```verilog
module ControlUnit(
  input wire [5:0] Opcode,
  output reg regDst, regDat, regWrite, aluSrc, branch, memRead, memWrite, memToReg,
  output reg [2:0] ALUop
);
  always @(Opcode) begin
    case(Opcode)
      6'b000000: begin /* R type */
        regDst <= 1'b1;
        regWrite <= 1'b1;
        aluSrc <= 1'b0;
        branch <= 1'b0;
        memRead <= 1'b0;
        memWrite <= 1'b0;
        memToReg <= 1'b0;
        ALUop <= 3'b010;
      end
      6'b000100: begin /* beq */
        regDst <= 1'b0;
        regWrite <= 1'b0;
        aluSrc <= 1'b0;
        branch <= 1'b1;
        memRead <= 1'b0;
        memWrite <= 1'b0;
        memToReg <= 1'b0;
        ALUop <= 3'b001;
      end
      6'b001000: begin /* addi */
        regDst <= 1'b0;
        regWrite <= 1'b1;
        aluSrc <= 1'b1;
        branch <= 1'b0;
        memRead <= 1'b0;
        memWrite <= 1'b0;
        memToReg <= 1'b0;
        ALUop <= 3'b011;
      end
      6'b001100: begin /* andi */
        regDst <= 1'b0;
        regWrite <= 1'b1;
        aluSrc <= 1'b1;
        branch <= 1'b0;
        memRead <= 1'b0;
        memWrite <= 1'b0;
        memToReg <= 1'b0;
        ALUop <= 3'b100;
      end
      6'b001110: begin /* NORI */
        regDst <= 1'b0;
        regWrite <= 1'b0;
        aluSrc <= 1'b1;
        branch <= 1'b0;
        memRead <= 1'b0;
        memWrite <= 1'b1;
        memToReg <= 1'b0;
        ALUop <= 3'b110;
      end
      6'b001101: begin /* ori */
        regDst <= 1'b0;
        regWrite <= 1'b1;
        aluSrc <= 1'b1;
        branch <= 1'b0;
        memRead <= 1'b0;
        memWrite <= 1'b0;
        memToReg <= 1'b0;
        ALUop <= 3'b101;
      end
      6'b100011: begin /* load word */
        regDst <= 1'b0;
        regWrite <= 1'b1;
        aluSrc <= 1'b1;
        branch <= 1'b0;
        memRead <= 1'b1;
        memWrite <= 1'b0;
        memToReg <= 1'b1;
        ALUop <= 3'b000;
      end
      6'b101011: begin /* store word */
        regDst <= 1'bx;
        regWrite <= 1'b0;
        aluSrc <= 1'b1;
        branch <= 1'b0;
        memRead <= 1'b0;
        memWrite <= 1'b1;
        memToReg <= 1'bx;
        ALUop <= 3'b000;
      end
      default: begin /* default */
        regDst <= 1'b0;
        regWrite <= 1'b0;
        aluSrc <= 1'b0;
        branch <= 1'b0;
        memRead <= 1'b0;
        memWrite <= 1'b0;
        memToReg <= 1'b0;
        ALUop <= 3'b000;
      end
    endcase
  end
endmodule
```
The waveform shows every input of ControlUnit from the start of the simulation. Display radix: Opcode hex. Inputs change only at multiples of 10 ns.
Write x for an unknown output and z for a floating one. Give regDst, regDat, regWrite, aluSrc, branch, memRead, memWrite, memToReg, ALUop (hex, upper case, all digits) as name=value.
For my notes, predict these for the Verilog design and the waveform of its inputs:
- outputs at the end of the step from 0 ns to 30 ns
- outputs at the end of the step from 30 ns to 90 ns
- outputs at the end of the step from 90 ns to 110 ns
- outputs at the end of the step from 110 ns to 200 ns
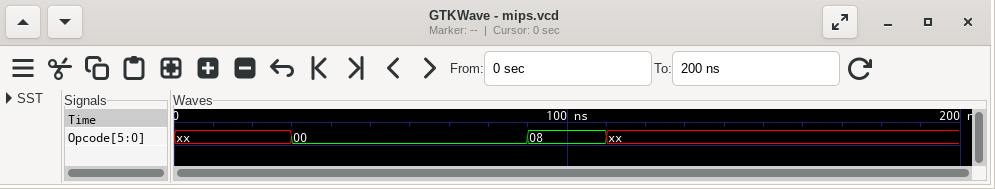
regDst=x, regDat=x, regWrite=x, aluSrc=x, branch=x, memRead=x, memWrite=x, memToReg=x, ALUop=x
regDst=1, regDat=x, regWrite=1, aluSrc=0, branch=0, memRead=0, memWrite=0, memToReg=0, ALUop=2
regDst=0, regDat=x, regWrite=1, aluSrc=1, branch=0, memRead=0, memWrite=0, memToReg=0, ALUop=3
regDst=0, regDat=x, regWrite=0, aluSrc=0, branch=0, memRead=0, memWrite=0, memToReg=0, ALUop=0
